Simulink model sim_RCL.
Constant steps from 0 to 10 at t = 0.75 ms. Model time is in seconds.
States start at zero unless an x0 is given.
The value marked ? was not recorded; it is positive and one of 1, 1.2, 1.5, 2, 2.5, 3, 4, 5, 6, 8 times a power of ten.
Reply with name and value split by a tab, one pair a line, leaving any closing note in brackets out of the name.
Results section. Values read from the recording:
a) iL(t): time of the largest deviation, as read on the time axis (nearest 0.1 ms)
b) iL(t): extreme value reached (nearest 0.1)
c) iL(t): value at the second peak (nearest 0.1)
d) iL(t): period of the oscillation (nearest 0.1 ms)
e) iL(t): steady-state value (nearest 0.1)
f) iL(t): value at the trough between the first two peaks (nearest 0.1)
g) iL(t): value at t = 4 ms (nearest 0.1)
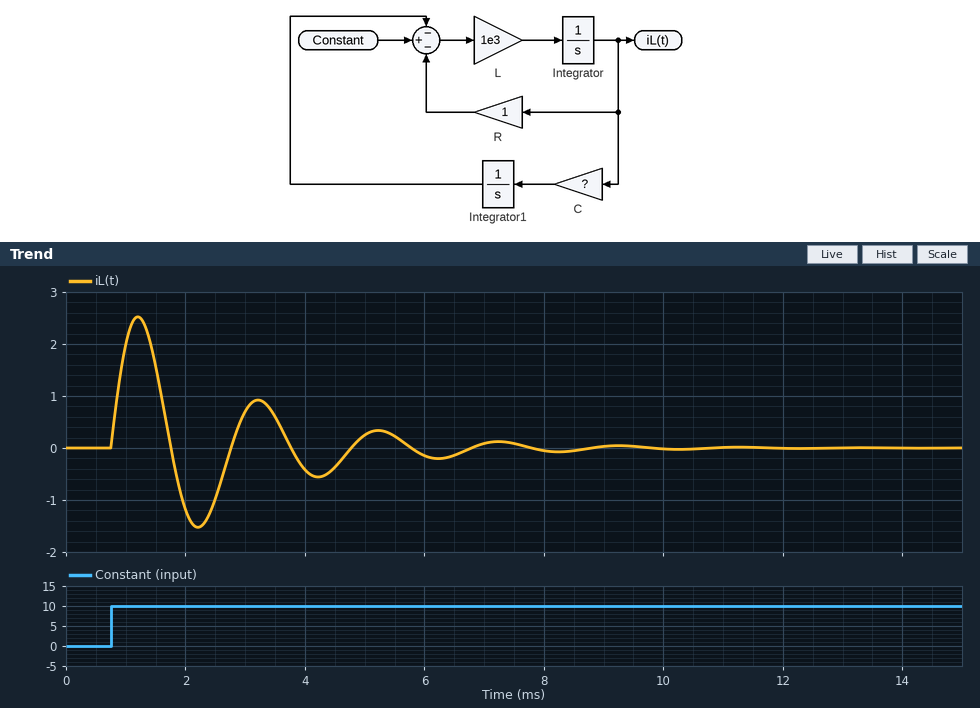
iL(t): time of the largest deviation, as read on the time axis	1.2 ms
iL(t): extreme value reached	2.5
iL(t): value at the second peak	0.9
iL(t): period of the oscillation	2.0 ms
iL(t): steady-state value	0.0
iL(t): value at the trough between the first two peaks	-1.5
iL(t): value at t = 4 ms	-0.4
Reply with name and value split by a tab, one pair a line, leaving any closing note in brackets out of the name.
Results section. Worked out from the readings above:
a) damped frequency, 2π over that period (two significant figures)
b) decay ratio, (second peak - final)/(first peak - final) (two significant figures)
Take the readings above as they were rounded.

damped frequency, 2π over that period	3.1 rad/ms
decay ratio, (second peak - final)/(first peak - final)	0.36
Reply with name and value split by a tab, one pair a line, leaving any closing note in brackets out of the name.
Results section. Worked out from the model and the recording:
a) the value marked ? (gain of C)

the value marked ?	10000
